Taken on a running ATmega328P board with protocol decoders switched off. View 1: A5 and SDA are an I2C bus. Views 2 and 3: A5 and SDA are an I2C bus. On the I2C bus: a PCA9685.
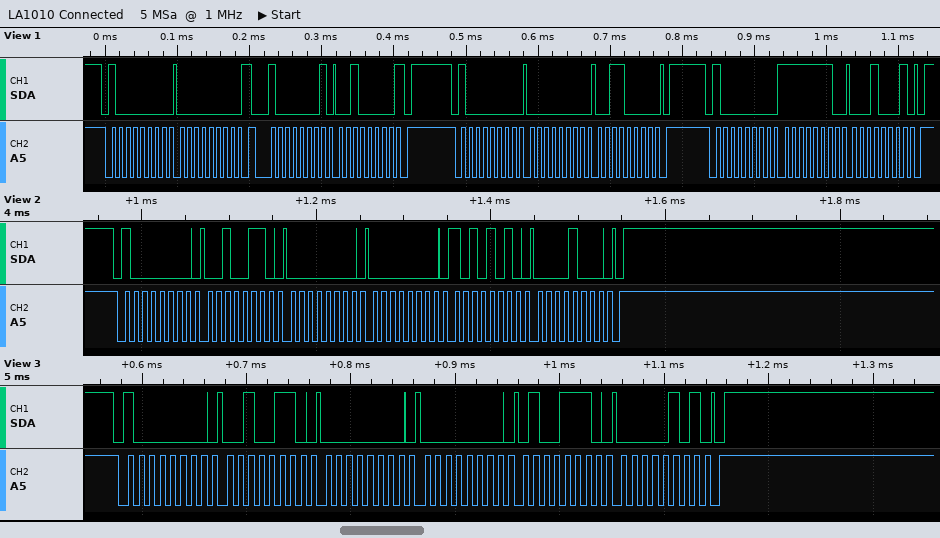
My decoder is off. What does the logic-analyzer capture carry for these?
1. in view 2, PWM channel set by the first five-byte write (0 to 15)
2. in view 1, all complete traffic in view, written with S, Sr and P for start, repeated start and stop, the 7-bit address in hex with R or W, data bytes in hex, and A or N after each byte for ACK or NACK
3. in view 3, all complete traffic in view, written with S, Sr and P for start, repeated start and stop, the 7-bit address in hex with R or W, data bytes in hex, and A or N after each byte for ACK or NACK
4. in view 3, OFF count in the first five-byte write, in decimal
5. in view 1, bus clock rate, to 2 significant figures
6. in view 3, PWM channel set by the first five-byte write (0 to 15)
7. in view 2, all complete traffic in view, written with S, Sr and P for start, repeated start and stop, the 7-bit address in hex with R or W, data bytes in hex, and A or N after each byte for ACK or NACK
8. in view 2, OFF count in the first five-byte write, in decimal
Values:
8
S 40W A 00 A Sr 40R A 20 N P S 40W A 00 A 30 A P S 40W A FE A 11 A P
S 40W A 26 A 00 A 00 A 4E A 05 A P
1358
100 kHz
8
S 40W A 26 A 00 A 00 A AA A 08 A P
2218
